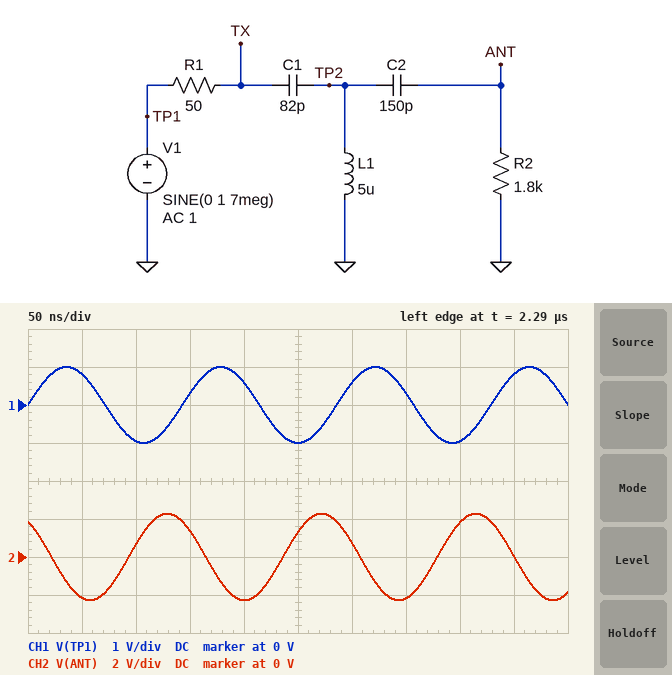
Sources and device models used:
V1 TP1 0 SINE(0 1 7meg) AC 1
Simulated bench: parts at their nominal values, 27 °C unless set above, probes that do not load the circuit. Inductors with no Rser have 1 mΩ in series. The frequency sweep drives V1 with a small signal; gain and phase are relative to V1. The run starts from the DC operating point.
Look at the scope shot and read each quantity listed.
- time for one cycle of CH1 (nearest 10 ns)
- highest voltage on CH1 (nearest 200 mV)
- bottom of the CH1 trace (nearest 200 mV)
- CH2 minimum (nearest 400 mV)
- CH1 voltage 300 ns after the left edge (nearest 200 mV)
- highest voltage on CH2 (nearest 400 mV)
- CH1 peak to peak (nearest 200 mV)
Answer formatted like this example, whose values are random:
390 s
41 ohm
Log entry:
140 ns
1.0 V
-1.0 V
-2.4 V
600 mV
2.4 V
2.0 V
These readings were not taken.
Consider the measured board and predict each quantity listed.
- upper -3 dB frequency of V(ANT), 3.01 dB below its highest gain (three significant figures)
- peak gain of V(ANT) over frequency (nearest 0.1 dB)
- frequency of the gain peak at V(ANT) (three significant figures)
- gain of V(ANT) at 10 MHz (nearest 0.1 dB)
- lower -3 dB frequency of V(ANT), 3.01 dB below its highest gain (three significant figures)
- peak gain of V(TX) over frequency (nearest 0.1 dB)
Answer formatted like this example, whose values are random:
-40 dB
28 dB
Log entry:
9.84 MHz
9.4 dB
7.94 MHz
6.1 dB
6.84 MHz
0 dB
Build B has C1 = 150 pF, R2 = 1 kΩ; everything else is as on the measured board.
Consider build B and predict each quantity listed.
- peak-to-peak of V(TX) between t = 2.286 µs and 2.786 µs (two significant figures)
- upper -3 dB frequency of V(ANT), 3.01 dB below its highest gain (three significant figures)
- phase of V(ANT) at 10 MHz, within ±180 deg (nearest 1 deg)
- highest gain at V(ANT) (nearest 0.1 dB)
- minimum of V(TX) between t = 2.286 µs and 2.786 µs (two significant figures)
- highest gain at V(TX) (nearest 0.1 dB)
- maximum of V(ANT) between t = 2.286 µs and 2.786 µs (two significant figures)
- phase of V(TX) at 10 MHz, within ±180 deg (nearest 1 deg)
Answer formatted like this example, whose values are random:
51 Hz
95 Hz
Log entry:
1.4 V
8.13 MHz
26 deg
6.8 dB
-690 mV
0 dB
1.9 V
11 deg
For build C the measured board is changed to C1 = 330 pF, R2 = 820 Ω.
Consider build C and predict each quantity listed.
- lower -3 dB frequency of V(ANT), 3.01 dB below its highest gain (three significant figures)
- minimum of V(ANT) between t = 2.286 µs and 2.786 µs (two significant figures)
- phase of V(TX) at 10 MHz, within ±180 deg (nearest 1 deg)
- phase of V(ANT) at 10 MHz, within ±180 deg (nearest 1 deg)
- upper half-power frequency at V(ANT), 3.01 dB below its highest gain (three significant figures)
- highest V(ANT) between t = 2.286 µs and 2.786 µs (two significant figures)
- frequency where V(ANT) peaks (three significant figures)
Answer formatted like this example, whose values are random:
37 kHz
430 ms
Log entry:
3.21 MHz
-1.2 V
9 deg
20 deg
6.41 MHz
1.2 V
4.03 MHz
